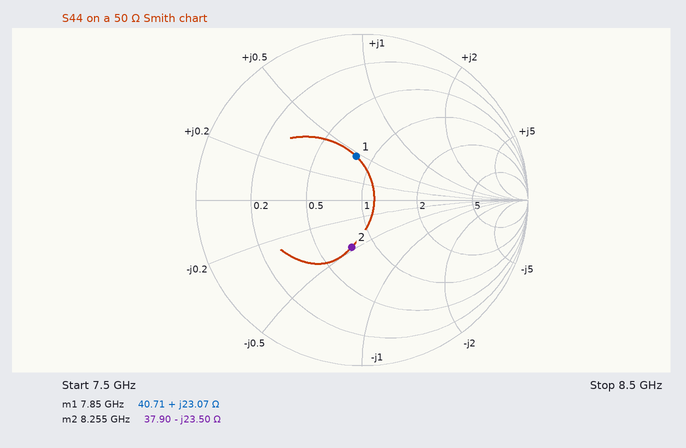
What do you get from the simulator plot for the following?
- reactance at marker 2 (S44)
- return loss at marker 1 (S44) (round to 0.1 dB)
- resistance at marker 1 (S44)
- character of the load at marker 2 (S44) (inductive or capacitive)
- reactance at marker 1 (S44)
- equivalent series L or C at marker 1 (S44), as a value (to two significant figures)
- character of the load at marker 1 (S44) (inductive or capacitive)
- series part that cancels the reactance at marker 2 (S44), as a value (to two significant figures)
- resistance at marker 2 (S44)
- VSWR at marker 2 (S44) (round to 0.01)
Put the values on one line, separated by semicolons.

-23.50 Ω; 11.5 dB; 40.71 Ω; capacitive; +23.07 Ω; 470 pH; inductive; 450 pH; 37.90 Ω; 1.82
